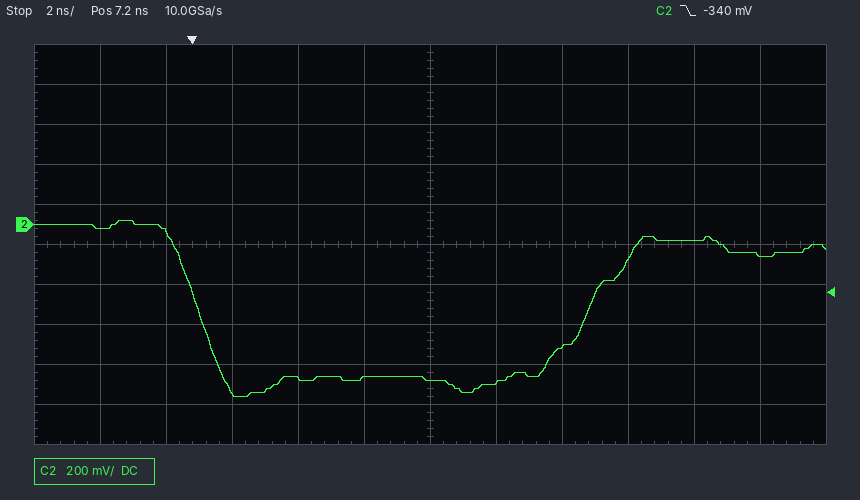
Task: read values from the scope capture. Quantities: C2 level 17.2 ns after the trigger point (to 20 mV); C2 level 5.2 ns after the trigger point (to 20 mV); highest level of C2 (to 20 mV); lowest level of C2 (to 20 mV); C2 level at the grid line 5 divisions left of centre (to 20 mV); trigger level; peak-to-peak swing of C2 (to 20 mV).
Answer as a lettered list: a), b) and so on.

a) -160 mV
b) -760 mV
c) 20 mV
d) -860 mV
e) -20 mV
f) -340 mV
g) 880 mV
